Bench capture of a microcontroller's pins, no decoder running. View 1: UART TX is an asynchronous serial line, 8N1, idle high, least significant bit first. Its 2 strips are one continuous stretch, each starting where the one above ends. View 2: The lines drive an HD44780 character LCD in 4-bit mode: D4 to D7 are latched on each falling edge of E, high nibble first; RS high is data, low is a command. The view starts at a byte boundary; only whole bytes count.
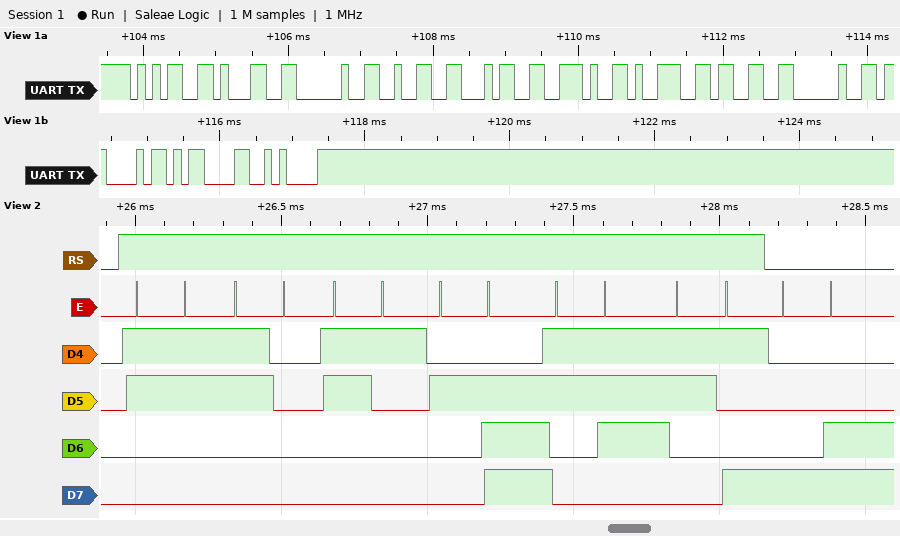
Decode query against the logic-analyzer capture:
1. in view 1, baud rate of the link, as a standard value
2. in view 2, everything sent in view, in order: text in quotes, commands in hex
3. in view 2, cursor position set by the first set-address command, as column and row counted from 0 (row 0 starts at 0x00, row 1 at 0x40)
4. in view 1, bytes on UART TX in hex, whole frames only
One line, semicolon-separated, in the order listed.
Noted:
9600 baud; "301.79" 0x8C; column 12, row 0; 0x35 0x31 0x20 0x32 0x34 0x2E 0x39 0x33 0x20 0x43 0x0D 0x0A
